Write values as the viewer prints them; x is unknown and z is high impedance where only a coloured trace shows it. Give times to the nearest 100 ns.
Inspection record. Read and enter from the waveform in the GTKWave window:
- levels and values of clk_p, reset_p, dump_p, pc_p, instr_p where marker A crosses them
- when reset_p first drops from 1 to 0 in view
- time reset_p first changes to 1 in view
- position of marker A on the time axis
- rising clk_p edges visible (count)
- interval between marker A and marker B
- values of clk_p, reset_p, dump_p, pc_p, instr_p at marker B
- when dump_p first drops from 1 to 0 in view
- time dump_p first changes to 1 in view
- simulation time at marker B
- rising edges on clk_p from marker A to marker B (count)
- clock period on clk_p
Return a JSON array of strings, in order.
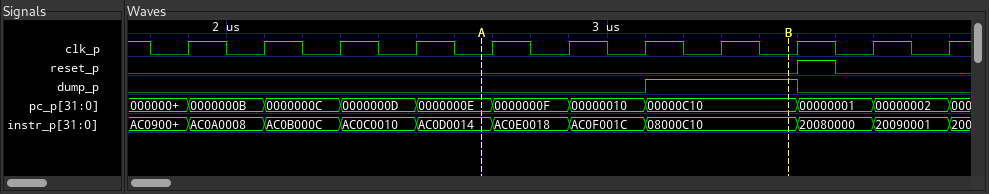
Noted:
["clk_p=0, reset_p=0, dump_p=0, pc_p=0000000E, instr_p=AC0D0014", "3600 ns", "3500 ns", "2700 ns", "11", "800 ns", "clk_p=0, reset_p=0, dump_p=1, pc_p=00000C10, instr_p=08000C10", "3500 ns", "3100 ns", "3500 ns", "4", "200 ns"]
